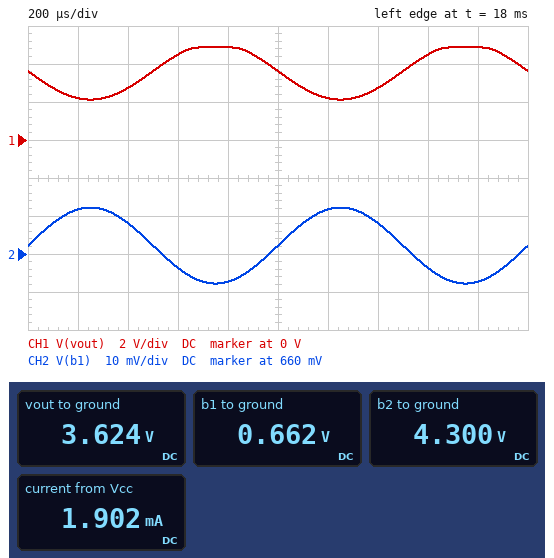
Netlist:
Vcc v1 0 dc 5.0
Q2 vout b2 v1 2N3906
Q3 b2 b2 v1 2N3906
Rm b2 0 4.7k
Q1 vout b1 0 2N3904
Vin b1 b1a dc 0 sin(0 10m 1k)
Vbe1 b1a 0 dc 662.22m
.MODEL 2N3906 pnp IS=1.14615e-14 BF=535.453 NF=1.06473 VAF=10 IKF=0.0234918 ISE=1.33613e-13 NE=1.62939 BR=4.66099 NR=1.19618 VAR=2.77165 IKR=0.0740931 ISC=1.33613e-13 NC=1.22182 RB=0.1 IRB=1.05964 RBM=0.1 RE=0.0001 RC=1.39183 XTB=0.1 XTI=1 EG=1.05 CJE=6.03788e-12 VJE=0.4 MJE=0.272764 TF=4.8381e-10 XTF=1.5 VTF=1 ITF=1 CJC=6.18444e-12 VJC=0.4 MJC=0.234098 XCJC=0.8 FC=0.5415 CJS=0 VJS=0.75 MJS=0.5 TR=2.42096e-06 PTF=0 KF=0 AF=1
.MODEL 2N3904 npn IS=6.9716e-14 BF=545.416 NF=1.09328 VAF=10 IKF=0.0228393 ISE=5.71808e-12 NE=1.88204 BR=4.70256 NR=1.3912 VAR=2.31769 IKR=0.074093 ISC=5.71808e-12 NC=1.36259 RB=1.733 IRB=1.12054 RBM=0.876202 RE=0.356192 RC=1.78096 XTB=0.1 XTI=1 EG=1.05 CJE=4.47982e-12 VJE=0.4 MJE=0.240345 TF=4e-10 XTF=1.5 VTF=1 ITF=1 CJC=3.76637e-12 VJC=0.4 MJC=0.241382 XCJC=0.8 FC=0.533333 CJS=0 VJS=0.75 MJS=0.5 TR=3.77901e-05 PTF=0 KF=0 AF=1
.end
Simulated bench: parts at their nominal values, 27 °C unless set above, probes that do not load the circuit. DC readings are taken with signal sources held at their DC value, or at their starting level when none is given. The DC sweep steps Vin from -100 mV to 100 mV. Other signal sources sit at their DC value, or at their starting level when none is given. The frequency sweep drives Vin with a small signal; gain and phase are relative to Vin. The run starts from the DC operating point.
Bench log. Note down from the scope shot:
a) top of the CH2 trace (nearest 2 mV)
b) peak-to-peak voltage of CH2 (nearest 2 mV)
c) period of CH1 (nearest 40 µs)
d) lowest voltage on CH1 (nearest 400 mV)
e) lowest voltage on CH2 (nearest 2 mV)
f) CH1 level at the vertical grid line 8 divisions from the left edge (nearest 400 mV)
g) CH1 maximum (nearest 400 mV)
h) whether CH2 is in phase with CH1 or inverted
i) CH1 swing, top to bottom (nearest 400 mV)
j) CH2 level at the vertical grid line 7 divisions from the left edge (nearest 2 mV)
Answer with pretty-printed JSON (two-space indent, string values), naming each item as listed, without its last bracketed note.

{
  "top of the CH2 trace": "672 mV",
  "peak-to-peak voltage of CH2": "20 mV",
  "period of CH1": "1.00 ms",
  "lowest voltage on CH1": "2.0 V",
  "lowest voltage on CH2": "652 mV",
  "CH1 level at the vertical grid line 8 divisions from the left edge": "4.4 V",
  "CH1 maximum": "4.8 V",
  "whether CH2 is in phase with CH1 or inverted": "inverted",
  "CH1 swing, top to bottom": "2.8 V",
  "CH2 level at the vertical grid line 7 divisions from the left edge": "668 mV"
}
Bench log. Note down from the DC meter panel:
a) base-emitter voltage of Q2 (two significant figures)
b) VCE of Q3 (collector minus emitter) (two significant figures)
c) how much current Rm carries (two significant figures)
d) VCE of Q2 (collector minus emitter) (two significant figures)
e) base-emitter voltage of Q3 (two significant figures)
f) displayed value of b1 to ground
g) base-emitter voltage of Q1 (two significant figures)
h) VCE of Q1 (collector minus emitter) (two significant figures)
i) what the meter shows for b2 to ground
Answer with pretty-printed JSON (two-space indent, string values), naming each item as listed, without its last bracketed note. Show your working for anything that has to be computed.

{
  "base-emitter voltage of Q2": "4.3 V - 5 V = -700 mV",
  "VCE of Q3 (collector minus emitter)": "4.3 V - 5 V = -700 mV",
  "how much current Rm carries": "(4.3 V) / 4.7 kΩ = 910 µA",
  "VCE of Q2 (collector minus emitter)": "3.624 V - 5 V = -1.4 V",
  "base-emitter voltage of Q3": "4.3 V - 5 V = -700 mV",
  "displayed value of b1 to ground": "0.662 V",
  "base-emitter voltage of Q1": "662 mV = 660 mV",
  "VCE of Q1 (collector minus emitter)": "3.624 V = 3.6 V",
  "what the meter shows for b2 to ground": "4.300 V"
}
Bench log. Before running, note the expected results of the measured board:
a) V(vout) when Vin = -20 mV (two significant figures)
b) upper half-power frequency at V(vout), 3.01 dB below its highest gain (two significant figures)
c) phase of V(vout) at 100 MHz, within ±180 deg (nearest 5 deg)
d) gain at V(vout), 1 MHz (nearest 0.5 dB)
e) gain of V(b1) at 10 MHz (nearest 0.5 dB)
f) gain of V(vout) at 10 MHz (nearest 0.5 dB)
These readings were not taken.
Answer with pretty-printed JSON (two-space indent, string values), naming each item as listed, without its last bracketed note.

{
  "V(vout) when Vin = -20 mV": "5.0 V",
  "upper half-power frequency at V(vout), 3.01 dB below its highest gain": "2.7 MHz",
  "phase of V(vout) at 100 MHz, within ±180 deg": "105 deg",
  "gain at V(vout), 1 MHz": "43.0 dB",
  "gain of V(b1) at 10 MHz": "0 dB",
  "gain of V(vout) at 10 MHz": "32.0 dB"
}
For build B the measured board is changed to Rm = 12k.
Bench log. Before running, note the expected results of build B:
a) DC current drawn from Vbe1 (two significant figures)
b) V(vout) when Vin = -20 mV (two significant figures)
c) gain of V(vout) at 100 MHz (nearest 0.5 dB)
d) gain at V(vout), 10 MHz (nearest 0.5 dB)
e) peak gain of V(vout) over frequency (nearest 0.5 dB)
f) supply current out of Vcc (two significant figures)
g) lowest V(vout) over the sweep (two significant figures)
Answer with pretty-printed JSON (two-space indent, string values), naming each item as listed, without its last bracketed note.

{
  "DC current drawn from Vbe1": "91 µA",
  "V(vout) when Vin = -20 mV": "2.4 V",
  "gain of V(vout) at 100 MHz": "-0.5 dB",
  "gain at V(vout), 10 MHz": "0 dB",
  "peak gain of V(vout) over frequency": "17.0 dB",
  "supply current out of Vcc": "920 µA",
  "lowest V(vout) over the sweep": "11 mV"
}
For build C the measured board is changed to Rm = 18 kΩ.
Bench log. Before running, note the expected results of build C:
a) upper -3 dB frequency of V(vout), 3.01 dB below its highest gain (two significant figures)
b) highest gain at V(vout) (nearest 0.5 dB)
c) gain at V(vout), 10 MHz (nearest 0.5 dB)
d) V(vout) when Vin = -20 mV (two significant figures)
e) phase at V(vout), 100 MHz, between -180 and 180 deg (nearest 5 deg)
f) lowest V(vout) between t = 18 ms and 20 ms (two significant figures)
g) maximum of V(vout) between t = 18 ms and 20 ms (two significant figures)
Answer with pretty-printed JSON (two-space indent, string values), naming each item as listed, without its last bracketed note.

{
  "upper -3 dB frequency of V(vout), 3.01 dB below its highest gain": "830 kHz",
  "highest gain at V(vout)": "5.0 dB",
  "gain at V(vout), 10 MHz": "-0.5 dB",
  "V(vout) when Vin = -20 mV": "580 mV",
  "phase at V(vout), 100 MHz, between -180 and 180 deg": "0 deg",
  "lowest V(vout) between t = 18 ms and 20 ms": "29 mV",
  "maximum of V(vout) between t = 18 ms and 20 ms": "70 mV"
}
